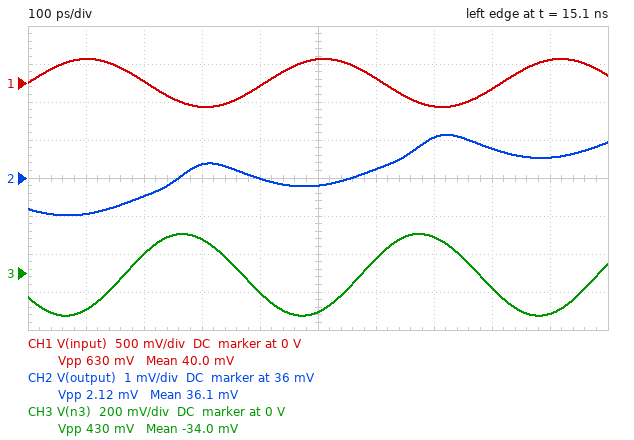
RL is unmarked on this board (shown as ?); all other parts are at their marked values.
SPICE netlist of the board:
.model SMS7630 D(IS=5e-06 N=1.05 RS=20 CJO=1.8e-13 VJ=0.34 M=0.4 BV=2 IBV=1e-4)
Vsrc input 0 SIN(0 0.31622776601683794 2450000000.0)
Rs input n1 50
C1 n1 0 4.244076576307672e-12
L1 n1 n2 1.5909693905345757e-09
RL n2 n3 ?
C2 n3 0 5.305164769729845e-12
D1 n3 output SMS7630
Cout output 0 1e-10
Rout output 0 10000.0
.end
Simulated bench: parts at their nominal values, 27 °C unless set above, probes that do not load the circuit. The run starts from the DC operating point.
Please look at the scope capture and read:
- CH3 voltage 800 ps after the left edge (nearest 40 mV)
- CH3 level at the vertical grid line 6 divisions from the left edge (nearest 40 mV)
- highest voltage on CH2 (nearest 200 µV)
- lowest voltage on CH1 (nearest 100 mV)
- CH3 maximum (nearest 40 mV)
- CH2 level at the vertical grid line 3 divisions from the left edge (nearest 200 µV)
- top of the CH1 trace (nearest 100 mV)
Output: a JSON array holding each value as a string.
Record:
["-80 mV", "80 mV", "37.2 mV", "-300 mV", "200 mV", "36.4 mV", "300 mV"]
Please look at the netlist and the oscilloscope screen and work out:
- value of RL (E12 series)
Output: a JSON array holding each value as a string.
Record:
["0.39 Ω"]
